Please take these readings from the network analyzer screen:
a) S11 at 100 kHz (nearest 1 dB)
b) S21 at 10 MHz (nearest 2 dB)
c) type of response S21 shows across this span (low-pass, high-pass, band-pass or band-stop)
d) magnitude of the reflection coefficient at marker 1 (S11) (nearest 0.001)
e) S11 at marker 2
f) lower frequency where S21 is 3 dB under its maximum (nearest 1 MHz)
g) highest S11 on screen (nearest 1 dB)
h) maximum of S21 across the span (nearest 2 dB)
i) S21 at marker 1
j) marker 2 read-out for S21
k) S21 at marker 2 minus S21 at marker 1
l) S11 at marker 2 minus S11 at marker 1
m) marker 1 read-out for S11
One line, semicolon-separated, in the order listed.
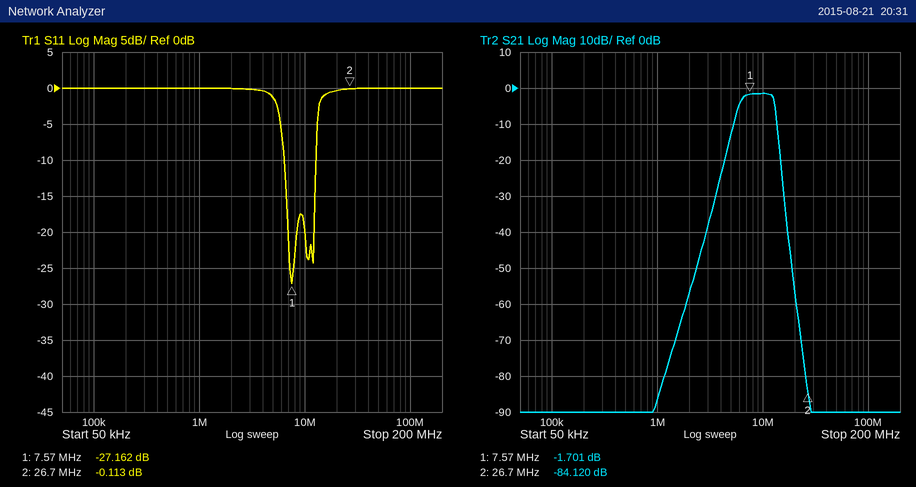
0 dB; -2 dB; band-pass; 0.044; -0.113 dB; 6 MHz; 0 dB; -2 dB; -1.701 dB; -84.120 dB; -82.419 dB; 27.049 dB; -27.162 dB
